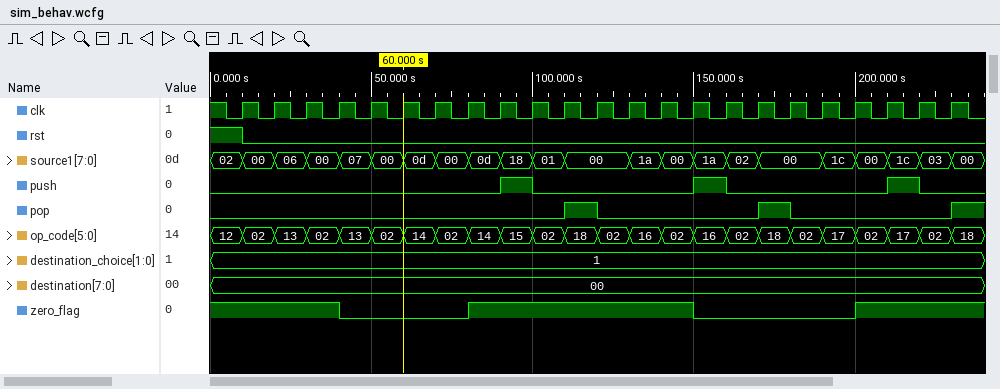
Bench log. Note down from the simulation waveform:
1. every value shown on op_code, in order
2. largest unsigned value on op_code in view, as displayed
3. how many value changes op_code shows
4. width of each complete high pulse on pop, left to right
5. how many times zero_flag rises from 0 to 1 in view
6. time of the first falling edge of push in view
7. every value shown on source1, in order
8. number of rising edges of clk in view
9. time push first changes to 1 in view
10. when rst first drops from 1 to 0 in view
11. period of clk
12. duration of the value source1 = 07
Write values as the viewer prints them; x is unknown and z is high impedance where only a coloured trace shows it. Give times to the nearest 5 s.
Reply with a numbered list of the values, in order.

1. 12, 02, 13, 02, 13, 02, 14, 02, 14, 15, 02, 18, 02, 16, 02, 16, 02, 18, 02, 17, 02, 17, 02, 18
2. 18
3. 23
4. 10 s, 10 s
5. 2
6. 100 s
7. 02, 00, 06, 00, 07, 00, 0d, 00, 0d, 18, 01, 00, 1a, 00, 1a, 02, 00, 1c, 00, 1c, 03, 00
8. 23
9. 90 s
10. 10 s
11. 10 s
12. 10 s
